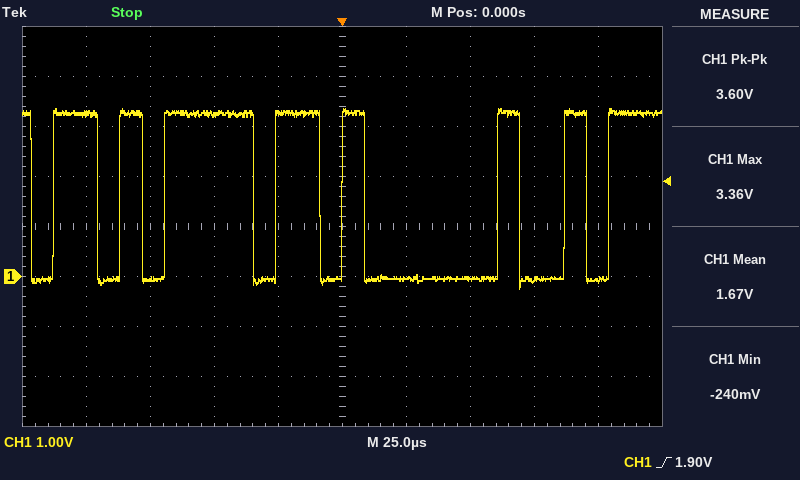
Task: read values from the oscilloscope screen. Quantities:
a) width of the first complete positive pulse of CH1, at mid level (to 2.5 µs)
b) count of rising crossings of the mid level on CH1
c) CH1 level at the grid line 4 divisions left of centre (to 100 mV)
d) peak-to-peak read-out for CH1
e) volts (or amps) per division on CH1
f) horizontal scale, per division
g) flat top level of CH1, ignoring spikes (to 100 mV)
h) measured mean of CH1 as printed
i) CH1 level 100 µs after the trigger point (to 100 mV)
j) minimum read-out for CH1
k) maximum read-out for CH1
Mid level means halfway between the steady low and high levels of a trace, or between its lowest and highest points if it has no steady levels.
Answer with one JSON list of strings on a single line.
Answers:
["17.5 µs", "8", "3.3 V", "3.60 V", "1 V", "25 µs", "3.3 V", "1.67 V", "-100 mV", "-240 mV", "3.36 V"]
